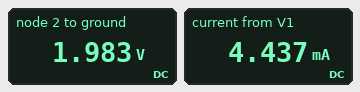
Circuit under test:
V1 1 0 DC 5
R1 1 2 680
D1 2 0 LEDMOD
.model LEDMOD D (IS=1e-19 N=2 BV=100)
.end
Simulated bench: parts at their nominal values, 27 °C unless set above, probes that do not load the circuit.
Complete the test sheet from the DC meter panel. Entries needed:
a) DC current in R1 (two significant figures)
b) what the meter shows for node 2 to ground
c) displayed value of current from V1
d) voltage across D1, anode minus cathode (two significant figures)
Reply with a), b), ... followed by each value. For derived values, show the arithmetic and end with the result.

a) (5 V - 1.983 V) / 680 Ω = 4.4 mA
b) 1.983 V
c) 4.437 mA
d) 1.983 V = 2.0 V
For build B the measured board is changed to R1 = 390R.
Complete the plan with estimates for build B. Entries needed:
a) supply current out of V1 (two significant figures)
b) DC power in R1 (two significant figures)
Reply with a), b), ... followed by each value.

a) 7.7 mA
b) 23 mW
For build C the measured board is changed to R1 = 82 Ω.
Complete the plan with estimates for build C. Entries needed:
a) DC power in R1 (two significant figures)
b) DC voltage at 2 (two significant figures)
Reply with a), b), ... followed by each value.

a) 100 mW
b) 2.1 V
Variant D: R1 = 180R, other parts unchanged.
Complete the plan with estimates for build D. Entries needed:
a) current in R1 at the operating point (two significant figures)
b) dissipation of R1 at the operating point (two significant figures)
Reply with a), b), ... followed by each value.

a) 16 mA
b) 48 mW
